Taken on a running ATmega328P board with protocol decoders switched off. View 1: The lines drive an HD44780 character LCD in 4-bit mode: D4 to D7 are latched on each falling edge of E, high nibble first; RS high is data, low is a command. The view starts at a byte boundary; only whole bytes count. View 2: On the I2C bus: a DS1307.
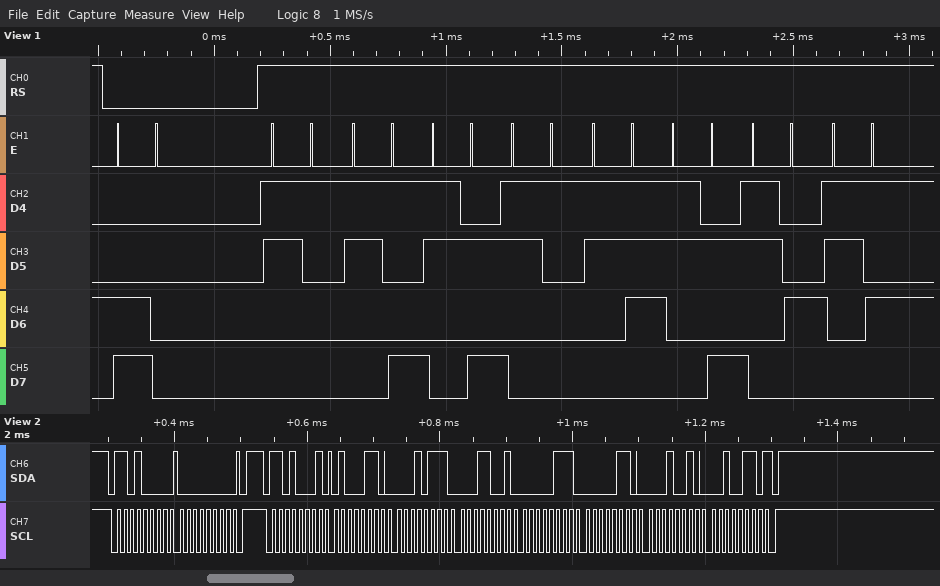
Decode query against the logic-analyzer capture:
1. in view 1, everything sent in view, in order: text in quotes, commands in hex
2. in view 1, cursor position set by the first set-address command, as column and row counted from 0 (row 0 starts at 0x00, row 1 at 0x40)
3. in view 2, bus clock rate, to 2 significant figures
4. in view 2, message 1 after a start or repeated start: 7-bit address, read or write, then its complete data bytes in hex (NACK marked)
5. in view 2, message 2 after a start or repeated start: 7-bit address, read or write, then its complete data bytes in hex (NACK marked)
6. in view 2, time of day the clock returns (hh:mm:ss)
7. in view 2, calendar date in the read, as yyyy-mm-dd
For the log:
0xC0 "19:17:45"
column 0, row 1
100 kHz
0x68 write: 00
0x68 read: 46 17 19 07 06 12 26 NACK
19:17:46
2026-12-06
